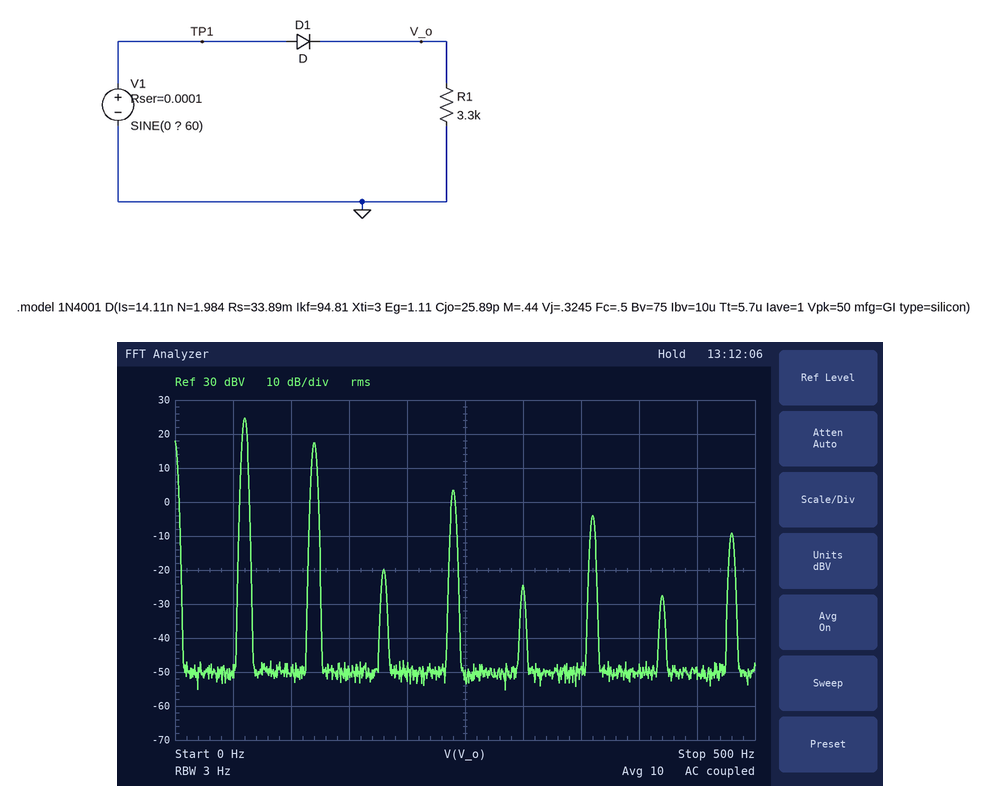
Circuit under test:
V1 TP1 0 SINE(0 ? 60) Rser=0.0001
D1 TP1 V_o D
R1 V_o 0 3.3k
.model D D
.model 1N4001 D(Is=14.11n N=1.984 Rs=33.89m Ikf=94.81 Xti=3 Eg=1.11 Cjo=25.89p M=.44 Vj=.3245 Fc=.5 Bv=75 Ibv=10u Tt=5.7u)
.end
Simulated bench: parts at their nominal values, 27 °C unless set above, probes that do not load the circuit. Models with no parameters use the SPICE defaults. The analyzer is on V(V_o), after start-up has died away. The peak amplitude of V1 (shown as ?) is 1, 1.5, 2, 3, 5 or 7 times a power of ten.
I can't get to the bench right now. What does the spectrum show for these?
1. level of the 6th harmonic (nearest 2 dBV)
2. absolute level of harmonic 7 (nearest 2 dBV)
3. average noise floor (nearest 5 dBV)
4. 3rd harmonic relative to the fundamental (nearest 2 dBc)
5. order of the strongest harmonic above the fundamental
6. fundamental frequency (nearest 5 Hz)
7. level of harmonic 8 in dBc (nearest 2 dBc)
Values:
-4 dBV
-28 dBV
-50 dBV
-44 dBc
2
60 Hz
-34 dBc
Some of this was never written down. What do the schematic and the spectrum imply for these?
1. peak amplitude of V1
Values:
50 V
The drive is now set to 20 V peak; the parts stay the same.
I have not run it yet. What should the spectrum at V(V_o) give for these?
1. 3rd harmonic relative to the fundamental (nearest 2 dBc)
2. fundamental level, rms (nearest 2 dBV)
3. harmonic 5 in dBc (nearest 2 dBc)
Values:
-36 dBc
16 dBV
-42 dBc
